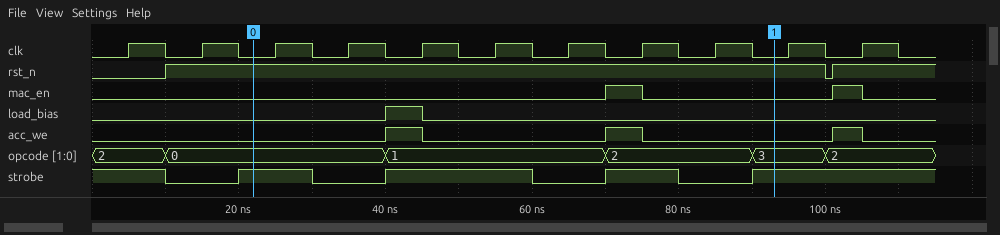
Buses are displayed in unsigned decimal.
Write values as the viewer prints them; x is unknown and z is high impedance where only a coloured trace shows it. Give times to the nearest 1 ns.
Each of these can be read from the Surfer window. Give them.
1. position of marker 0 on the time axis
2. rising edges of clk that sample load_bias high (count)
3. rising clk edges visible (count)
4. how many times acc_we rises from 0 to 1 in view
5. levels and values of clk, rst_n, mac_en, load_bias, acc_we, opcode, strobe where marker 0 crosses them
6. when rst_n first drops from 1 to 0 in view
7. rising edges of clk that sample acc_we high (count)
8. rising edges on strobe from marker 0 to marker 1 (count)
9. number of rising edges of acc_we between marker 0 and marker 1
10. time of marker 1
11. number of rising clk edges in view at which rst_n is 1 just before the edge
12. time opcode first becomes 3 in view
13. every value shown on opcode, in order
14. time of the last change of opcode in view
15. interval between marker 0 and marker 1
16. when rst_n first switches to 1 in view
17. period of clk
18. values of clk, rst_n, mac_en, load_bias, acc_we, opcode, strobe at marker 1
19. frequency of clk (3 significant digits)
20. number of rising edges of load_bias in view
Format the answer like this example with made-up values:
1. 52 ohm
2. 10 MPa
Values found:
1. 22 ns
2. 1
3. 11
4. 3
5. clk=0, rst_n=1, mac_en=0, load_bias=0, acc_we=0, opcode=0, strobe=1
6. 100 ns
7. 3
8. 3
9. 2
10. 93 ns
11. 10
12. 90 ns
13. 2, 0, 1, 2, 3, 2
14. 100 ns
15. 71 ns
16. 10 ns
17. 10 ns
18. clk=0, rst_n=1, mac_en=0, load_bias=0, acc_we=0, opcode=3, strobe=1
19. 100 MHz
20. 1
